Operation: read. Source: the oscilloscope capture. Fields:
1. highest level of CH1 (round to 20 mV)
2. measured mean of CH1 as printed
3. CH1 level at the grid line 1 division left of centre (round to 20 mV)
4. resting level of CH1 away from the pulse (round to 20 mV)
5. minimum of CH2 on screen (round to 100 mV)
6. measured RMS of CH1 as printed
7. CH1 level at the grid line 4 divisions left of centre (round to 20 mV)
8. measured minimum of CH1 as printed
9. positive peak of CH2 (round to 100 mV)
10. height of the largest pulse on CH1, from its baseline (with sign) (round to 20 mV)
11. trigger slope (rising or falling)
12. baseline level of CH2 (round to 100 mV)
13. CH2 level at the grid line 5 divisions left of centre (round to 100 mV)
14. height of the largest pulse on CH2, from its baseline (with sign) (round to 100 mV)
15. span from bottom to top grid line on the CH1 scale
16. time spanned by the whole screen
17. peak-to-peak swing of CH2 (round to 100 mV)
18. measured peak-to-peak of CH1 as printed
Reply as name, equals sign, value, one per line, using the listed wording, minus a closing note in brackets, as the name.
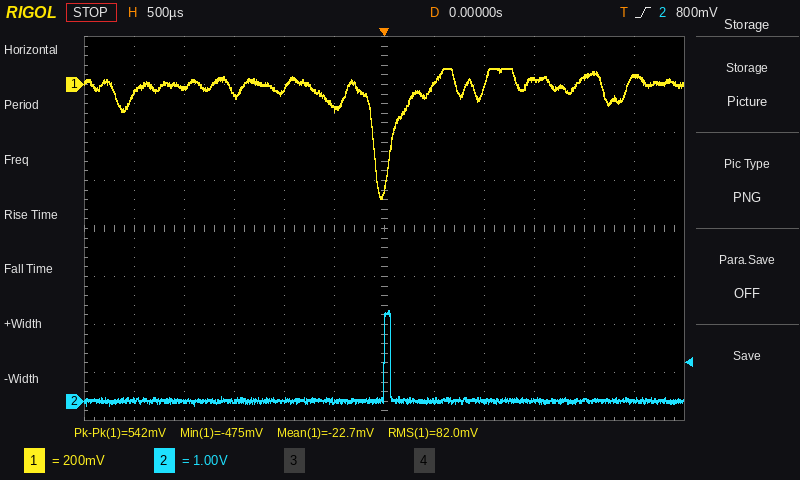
highest level of CH1 = 60 mV
measured mean of CH1 as printed = -22.7 mV
CH1 level at the grid line 1 division left of centre = -100 mV
resting level of CH1 away from the pulse = 0 mV
minimum of CH2 on screen = -100 mV
measured RMS of CH1 as printed = 82.0 mV
CH1 level at the grid line 4 divisions left of centre = -20 mV
measured minimum of CH1 as printed = -475 mV
positive peak of CH2 = 1.9 V
height of the largest pulse on CH1, from its baseline (with sign) = -480 mV
trigger slope = rising
baseline level of CH2 = 0.0 V
CH2 level at the grid line 5 divisions left of centre = 0.0 V
height of the largest pulse on CH2, from its baseline (with sign) = +1.9 V
span from bottom to top grid line on the CH1 scale = 1.6 V
time spanned by the whole screen = 6 ms
peak-to-peak swing of CH2 = 2.0 V
measured peak-to-peak of CH1 as printed = 542 mV
